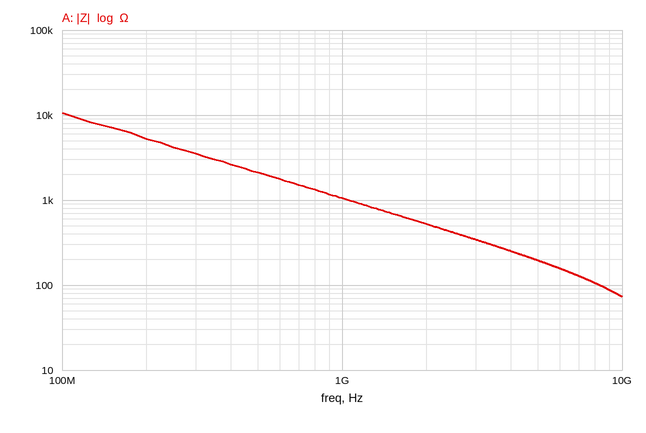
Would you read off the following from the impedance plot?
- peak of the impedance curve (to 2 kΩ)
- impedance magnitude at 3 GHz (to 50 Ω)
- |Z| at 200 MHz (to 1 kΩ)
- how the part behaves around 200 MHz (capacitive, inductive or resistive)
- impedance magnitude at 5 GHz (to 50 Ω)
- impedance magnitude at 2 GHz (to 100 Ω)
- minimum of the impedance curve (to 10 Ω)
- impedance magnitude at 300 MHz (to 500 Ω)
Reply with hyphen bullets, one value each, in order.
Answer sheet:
- 10 kΩ
- 350 Ω
- 5 kΩ
- capacitive
- 200 Ω
- 500 Ω
- 70 Ω
- 3.5 kΩ
